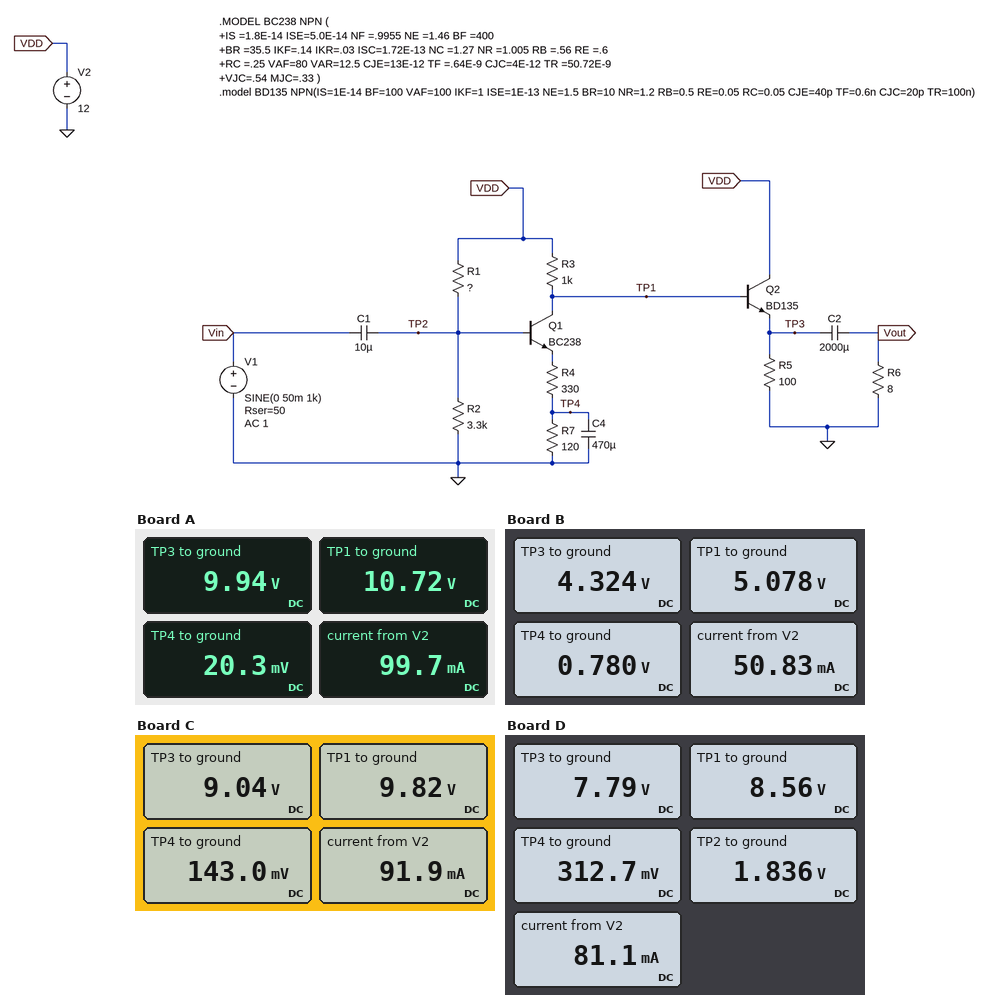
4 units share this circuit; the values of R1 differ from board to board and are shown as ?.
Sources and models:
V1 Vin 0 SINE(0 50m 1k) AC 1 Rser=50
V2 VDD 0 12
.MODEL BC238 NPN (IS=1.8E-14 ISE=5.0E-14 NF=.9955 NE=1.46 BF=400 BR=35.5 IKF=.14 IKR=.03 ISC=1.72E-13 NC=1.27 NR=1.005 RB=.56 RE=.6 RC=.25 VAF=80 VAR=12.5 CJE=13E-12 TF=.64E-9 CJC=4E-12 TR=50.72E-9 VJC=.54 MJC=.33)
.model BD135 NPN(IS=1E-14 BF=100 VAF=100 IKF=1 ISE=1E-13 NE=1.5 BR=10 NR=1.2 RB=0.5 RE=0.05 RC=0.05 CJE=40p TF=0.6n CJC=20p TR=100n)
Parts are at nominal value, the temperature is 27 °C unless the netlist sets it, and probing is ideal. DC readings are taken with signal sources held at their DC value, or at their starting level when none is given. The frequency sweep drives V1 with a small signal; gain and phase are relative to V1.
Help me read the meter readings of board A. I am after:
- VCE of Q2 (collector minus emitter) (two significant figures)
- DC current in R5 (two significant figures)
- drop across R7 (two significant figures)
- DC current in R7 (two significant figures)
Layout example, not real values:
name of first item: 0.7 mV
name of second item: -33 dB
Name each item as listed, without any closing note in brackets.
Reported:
VCE of Q2 (collector minus emitter): 2.1 V
DC current in R5: 99 mA
drop across R7: 20 mV
DC current in R7: 170 µA
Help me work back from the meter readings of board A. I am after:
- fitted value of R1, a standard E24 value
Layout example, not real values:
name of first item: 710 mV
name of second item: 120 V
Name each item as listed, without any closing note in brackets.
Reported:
fitted value of R1, a standard E24 value: 56 kΩ
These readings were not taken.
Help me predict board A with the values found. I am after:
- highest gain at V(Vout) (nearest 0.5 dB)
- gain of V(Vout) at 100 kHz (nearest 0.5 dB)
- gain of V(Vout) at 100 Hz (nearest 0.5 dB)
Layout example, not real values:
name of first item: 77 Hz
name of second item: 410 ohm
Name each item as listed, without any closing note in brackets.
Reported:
highest gain at V(Vout): -2.5 dB
gain of V(Vout) at 100 kHz: -2.5 dB
gain of V(Vout) at 100 Hz: -2.5 dB
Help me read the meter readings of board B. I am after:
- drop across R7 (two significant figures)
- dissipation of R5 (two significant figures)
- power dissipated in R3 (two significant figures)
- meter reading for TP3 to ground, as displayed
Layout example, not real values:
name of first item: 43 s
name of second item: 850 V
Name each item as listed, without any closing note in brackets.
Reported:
drop across R7: 780 mV
dissipation of R5: 190 mW
power dissipated in R3: 48 mW
meter reading for TP3 to ground, as displayed: 4.324 V
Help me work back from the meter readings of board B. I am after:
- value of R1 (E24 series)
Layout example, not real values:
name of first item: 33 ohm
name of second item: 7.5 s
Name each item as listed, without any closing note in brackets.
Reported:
value of R1: 7.5 kΩ
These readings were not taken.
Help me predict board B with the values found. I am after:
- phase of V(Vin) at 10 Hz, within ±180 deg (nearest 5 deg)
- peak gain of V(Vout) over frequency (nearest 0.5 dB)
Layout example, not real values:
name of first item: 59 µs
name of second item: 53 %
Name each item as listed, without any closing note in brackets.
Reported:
phase of V(Vin) at 10 Hz, within ±180 deg: 0 deg
peak gain of V(Vout) over frequency: 1.5 dB
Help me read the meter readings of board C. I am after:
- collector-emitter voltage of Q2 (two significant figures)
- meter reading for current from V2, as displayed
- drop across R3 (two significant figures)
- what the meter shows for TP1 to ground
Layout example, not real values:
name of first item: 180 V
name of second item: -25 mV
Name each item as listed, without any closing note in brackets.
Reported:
collector-emitter voltage of Q2: 3.0 V
meter reading for current from V2, as displayed: 91.9 mA
drop across R3: 2.2 V
what the meter shows for TP1 to ground: 9.82 V
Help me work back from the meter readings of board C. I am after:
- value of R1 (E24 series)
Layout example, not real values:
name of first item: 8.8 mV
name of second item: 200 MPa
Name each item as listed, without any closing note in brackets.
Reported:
value of R1: 30 kΩ
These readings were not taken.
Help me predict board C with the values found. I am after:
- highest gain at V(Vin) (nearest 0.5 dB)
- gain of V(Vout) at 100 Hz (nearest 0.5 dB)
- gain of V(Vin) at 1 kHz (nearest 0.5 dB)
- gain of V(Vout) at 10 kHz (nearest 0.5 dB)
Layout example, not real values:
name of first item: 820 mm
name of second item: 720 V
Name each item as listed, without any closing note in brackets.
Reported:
highest gain at V(Vin): 0 dB
gain of V(Vout) at 100 Hz: 0.5 dB
gain of V(Vin) at 1 kHz: 0 dB
gain of V(Vout) at 10 kHz: 0.5 dB
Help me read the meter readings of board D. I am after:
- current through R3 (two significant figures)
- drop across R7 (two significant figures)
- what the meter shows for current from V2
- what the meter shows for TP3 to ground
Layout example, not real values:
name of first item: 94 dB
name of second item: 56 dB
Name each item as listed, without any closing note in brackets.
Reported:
current through R3: 3.4 mA
drop across R7: 310 mV
what the meter shows for current from V2: 81.1 mA
what the meter shows for TP3 to ground: 7.79 V
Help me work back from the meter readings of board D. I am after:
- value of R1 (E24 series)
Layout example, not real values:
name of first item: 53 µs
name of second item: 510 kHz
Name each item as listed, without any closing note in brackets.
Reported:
value of R1: 18 kΩ
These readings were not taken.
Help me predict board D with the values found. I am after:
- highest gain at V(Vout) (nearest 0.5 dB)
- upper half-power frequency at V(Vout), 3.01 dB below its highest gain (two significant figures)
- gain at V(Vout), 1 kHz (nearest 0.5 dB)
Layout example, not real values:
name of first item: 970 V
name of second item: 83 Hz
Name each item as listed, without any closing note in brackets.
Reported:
highest gain at V(Vout): 1.0 dB
upper half-power frequency at V(Vout), 3.01 dB below its highest gain: 4.2 MHz
gain at V(Vout), 1 kHz: 1.0 dB
